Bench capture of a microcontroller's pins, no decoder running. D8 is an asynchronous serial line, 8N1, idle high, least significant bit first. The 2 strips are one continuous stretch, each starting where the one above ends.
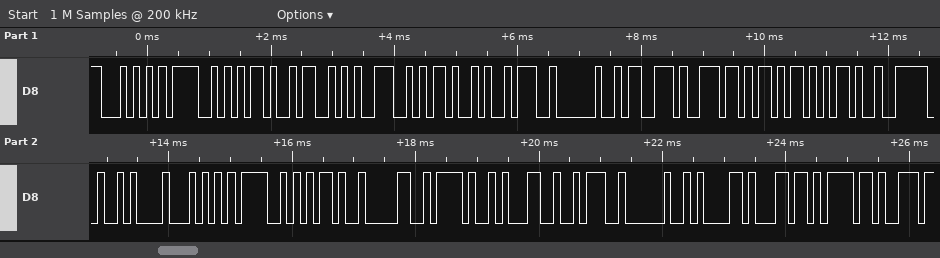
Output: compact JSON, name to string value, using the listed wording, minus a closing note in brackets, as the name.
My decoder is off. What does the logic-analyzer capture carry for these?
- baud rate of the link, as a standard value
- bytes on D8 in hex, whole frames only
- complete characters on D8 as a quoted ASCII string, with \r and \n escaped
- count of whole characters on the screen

{"baud rate of the link, as a standard value": "9600 baud", "bytes on D8 in hex, whole frames only": "0x54 0x4F 0x2D 0x53 0x4E 0x4B 0x3A 0x20 0x73 0x6E 0x6B 0x2D 0x3E 0x0A 0x54 0x4F 0x2D 0x30 0x2F 0x31 0x3A 0x20 0x61 0x6C 0x6F", "complete characters on D8 as a quoted ASCII string, with \\r and \\n escaped": "\"TO-SNK: snk->\\nTO-0/1: alo\"", "count of whole characters on the screen": "25"}
